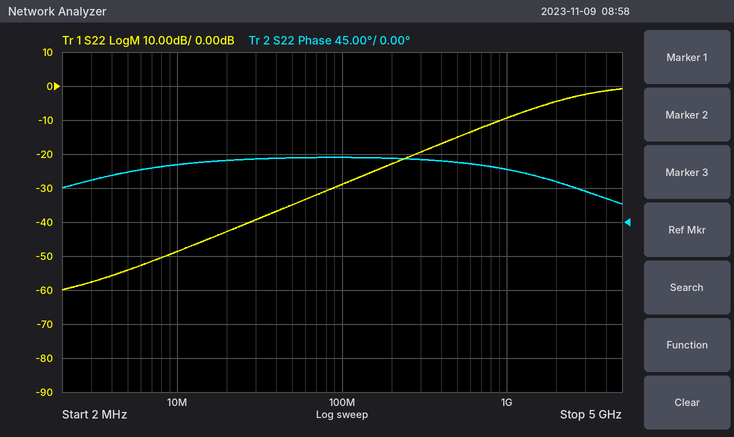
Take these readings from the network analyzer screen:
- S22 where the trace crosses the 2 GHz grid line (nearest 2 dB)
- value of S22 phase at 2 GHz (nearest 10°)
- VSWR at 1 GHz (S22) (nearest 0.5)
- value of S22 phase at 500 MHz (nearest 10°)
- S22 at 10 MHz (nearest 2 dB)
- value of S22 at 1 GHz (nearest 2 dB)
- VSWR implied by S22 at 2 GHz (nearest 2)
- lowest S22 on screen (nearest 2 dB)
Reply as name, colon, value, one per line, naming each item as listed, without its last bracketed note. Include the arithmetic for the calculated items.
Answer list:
S22 where the trace crosses the 2 GHz grid line: -4 dB
value of S22 phase at 2 GHz: 50°
VSWR at 1 GHz (S22): |Γ| = 10^(-10/20) = 0.3162; VSWR = (1 + 0.3162)/(1 − 0.3162) ≈ 1.92, so 2.0 to the nearest 0.5
value of S22 phase at 500 MHz: 80°
S22 at 10 MHz: -48 dB
value of S22 at 1 GHz: -10 dB
VSWR implied by S22 at 2 GHz: |Γ| = 10^(-4/20) = 0.6310; VSWR = (1 + 0.6310)/(1 − 0.6310) ≈ 4
lowest S22 on screen: -60 dB
